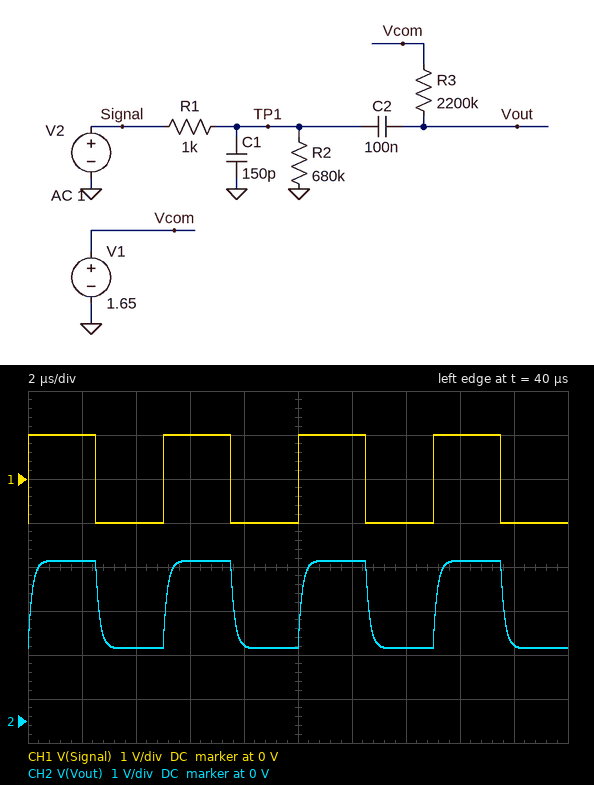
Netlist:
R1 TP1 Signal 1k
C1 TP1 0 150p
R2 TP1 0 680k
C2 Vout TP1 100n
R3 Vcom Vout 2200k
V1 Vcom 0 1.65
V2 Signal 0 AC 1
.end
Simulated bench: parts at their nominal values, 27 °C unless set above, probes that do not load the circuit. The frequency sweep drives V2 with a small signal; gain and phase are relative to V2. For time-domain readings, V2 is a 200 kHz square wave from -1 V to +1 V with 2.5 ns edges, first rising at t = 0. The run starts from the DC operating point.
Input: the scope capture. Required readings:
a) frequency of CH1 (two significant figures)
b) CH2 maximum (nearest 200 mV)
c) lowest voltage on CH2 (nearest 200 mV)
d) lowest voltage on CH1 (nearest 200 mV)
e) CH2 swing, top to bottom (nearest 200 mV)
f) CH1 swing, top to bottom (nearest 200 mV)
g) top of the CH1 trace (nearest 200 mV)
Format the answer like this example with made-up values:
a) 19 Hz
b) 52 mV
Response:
a) 200 kHz
b) 3.6 V
c) 1.6 V
d) -1.0 V
e) 2.0 V
f) 2.0 V
g) 1.0 V
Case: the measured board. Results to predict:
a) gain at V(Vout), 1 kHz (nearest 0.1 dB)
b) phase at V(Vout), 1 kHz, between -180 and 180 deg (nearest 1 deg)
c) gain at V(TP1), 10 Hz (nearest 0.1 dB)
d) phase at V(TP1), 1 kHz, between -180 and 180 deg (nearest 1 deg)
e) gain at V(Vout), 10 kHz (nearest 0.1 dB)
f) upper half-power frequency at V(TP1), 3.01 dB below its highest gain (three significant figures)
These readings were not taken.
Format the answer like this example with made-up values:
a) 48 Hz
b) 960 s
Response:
a) 0 dB
b) 0 deg
c) 0 dB
d) 0 deg
e) 0 dB
f) 1.06 MHz
